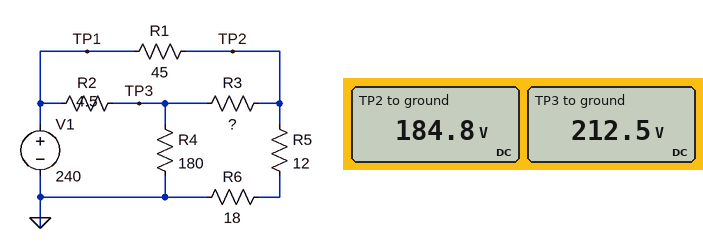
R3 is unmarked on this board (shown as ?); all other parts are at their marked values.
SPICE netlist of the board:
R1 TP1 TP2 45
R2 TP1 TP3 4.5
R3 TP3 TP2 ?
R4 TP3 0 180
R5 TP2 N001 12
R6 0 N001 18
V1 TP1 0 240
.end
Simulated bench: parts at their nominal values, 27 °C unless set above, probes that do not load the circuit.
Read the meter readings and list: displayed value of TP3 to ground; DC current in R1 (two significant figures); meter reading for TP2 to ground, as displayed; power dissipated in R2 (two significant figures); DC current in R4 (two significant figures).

212.5 V
1.2 A
184.8 V
170 W
1.2 A
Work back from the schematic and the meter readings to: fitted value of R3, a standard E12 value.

5.6 Ω
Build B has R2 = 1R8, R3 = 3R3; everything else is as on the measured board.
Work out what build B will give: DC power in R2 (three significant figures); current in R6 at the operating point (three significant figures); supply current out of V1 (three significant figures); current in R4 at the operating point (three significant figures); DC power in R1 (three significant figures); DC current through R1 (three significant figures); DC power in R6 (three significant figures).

98.4 W
6.88 A
8.14 A
1.26 A
25.0 W
746 mA
852 W
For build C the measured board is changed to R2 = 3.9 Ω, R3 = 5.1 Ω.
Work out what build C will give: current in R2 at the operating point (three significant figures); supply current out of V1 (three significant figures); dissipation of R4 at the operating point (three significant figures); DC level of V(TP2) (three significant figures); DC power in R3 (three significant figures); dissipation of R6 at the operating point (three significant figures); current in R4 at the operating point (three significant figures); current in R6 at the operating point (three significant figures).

6.36 A
7.49 A
257 W
189 V
136 W
714 W
1.20 A
6.30 A
